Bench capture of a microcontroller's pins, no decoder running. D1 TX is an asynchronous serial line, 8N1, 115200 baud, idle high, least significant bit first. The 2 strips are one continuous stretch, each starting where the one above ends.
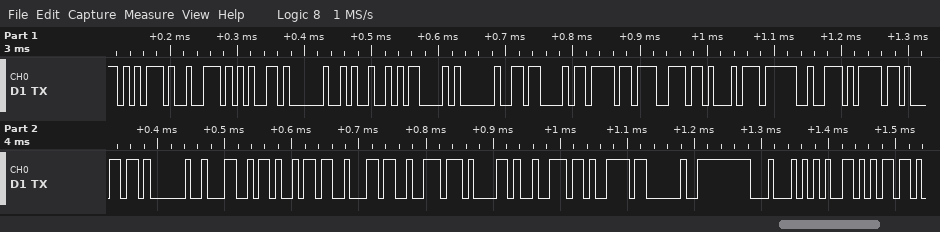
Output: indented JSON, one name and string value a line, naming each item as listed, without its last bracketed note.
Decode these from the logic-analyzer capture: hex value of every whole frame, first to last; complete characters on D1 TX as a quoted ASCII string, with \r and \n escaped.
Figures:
{
  "hex value of every whole frame, first to last": "75 72 65 20 49 43 20 43 6F 6E 74 72 6F 6C 20 4C 69 62 72 61 72 79 20 44 65 6D",
  "complete characters on D1 TX as a quoted ASCII string, with \\r and \\n escaped": "\"ure IC Control Library Dem\""
}
